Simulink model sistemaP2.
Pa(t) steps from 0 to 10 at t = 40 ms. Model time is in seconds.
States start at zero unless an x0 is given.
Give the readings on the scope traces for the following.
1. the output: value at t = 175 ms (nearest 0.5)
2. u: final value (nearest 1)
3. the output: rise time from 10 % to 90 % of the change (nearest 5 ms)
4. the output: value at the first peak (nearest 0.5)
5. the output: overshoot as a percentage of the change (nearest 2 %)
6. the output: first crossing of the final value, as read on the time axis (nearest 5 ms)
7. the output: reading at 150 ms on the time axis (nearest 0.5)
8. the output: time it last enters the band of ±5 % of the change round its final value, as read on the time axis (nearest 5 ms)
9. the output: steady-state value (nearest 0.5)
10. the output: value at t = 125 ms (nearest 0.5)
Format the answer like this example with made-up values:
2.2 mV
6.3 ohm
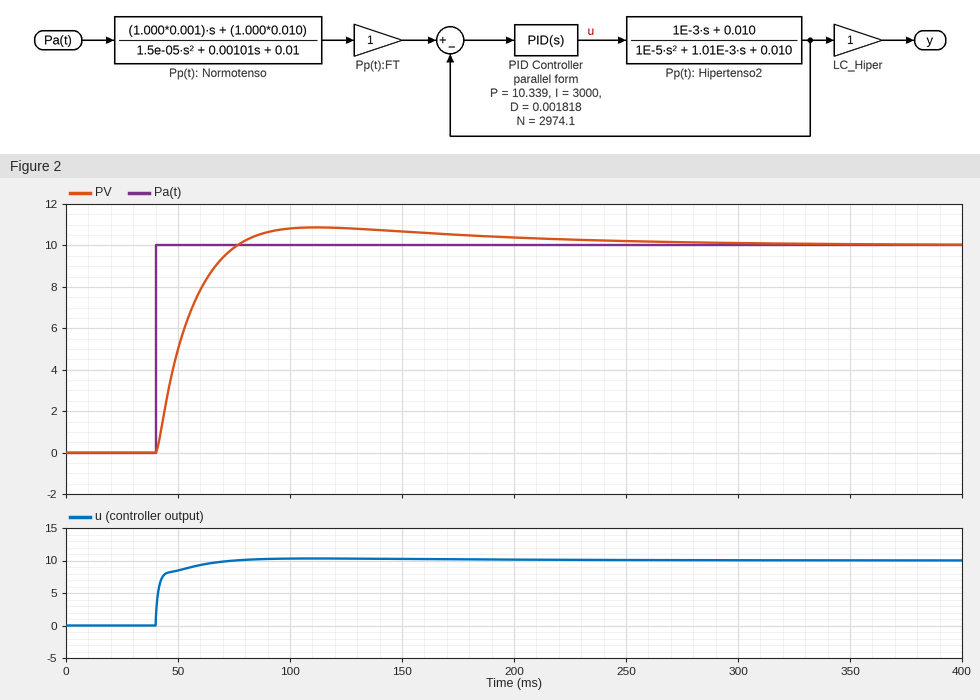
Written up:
10.5
10
25 ms
11.0
8 %
75 ms
10.5
175 ms
10.0
11.0
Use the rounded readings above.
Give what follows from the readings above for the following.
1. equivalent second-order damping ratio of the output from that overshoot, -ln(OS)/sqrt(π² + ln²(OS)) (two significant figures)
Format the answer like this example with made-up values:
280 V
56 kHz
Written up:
0.63
